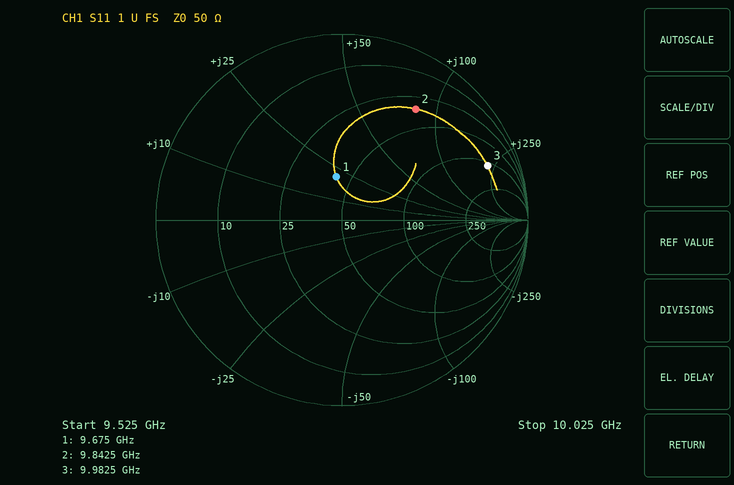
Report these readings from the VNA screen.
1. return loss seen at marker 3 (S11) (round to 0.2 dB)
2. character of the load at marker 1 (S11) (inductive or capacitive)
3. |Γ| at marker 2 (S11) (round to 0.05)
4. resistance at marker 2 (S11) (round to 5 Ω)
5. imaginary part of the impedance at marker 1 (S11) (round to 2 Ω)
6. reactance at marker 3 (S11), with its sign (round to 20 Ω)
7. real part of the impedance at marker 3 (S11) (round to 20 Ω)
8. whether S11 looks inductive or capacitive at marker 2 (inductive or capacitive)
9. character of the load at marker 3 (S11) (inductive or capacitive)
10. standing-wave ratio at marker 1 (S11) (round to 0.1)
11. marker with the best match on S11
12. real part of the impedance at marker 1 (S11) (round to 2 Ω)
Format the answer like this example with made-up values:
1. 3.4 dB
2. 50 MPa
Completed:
1. 1.6 dB
2. inductive
3. 0.70
4. 35 Ω
5. +20 Ω
6. +220 Ω
7. 120 Ω
8. inductive
9. inductive
10. 1.6
11. marker 1
12. 42 Ω
